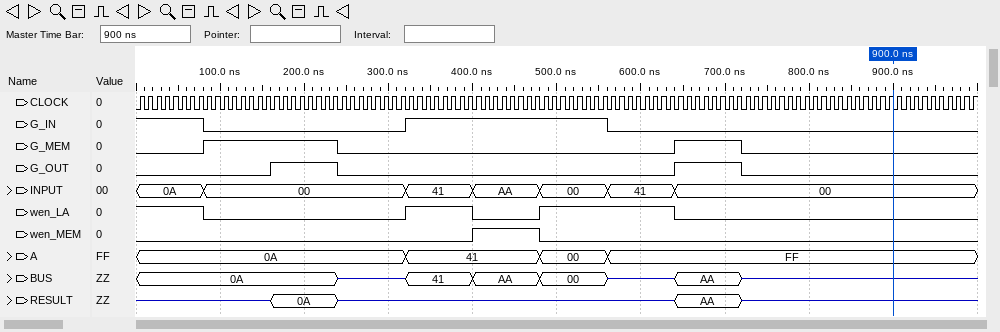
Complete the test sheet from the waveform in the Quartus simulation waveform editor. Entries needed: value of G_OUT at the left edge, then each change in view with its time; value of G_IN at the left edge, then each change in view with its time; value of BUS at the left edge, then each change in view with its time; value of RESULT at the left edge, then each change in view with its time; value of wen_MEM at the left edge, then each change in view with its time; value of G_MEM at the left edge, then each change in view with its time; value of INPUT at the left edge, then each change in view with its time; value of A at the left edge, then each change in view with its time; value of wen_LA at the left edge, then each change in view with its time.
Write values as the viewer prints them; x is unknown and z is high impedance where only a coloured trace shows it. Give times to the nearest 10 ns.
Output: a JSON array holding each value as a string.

["0, 1 at 160 ns, 0 at 240 ns, 1 at 640 ns, 0 at 720 ns", "1, 0 at 80 ns, 1 at 320 ns, 0 at 560 ns", "0A, z at 240 ns, 41 at 320 ns, AA at 400 ns, 00 at 480 ns, z at 560 ns, AA at 640 ns, z at 720 ns", "z, 0A at 160 ns, z at 240 ns, AA at 640 ns, z at 720 ns", "0, 1 at 400 ns, 0 at 480 ns", "0, 1 at 80 ns, 0 at 240 ns, 1 at 640 ns, 0 at 720 ns", "0A, 00 at 80 ns, 41 at 320 ns, AA at 400 ns, 00 at 480 ns, 41 at 560 ns, 00 at 640 ns", "0A, 41 at 320 ns, 00 at 480 ns, FF at 560 ns", "1, 0 at 80 ns, 1 at 320 ns, 0 at 400 ns, 1 at 480 ns, 0 at 640 ns"]
